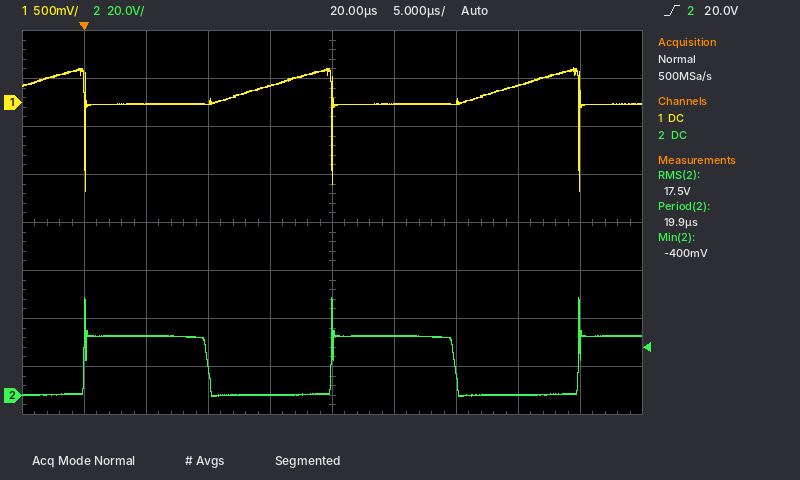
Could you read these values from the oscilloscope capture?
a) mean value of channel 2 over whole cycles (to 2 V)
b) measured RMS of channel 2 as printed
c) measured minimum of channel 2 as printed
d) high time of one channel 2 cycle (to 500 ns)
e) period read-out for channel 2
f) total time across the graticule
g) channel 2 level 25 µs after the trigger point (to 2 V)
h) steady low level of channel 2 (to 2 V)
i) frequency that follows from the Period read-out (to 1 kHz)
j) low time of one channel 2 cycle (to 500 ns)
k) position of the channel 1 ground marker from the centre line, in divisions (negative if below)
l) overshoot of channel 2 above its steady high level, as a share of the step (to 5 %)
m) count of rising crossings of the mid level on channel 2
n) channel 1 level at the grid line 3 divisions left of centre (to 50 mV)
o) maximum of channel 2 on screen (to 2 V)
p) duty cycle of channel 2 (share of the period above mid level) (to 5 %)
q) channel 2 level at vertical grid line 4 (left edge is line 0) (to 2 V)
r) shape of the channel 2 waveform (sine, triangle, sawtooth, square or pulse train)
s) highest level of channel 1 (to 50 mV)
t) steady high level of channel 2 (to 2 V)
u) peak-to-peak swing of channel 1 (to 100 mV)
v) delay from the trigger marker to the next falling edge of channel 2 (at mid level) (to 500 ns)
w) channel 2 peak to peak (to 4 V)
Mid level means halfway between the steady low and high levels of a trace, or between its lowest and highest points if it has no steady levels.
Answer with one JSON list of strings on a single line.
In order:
["12 V", "17.5 V", "-400 mV", "10.0 µs", "19.9 µs", "50 µs", "24 V", "0 V", "50 kHz", "10.0 µs", "+2.5 div", "65 %", "3", "0 mV", "40 V", "50 %", "0 V", "square", "350 mV", "24 V", "1.30 V", "10.0 µs", "40 V"]
